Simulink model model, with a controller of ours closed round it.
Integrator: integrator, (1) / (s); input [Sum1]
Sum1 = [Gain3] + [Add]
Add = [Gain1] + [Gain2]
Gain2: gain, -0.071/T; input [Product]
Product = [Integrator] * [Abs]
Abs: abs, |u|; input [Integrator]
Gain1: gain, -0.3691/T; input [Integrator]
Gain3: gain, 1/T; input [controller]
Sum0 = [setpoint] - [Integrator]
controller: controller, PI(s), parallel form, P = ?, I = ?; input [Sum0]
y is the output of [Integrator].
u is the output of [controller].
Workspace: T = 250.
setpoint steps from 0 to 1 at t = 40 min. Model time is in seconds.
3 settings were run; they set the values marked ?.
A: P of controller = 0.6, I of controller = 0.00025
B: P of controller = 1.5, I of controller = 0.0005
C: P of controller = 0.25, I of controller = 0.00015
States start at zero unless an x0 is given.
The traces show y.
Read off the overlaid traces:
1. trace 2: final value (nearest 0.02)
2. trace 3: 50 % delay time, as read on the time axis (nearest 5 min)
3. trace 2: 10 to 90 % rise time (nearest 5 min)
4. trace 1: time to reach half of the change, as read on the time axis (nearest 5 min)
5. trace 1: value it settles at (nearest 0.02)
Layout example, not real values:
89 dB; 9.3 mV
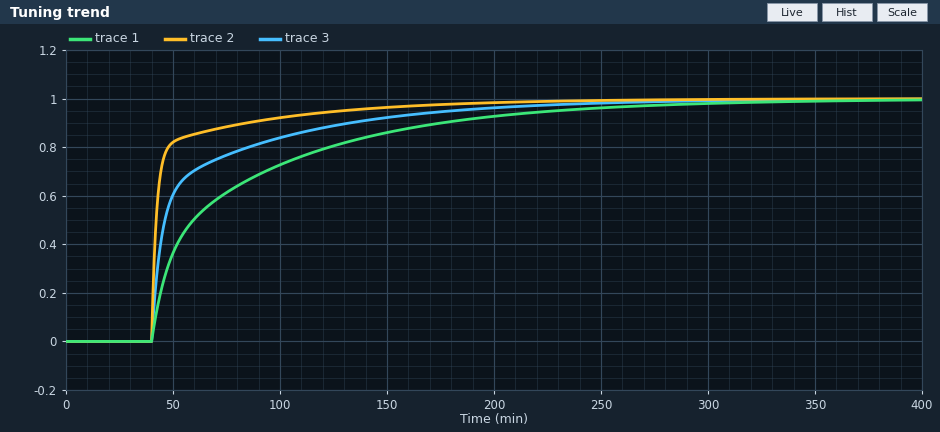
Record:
1.00; 45 min; 45 min; 60 min; 1.00
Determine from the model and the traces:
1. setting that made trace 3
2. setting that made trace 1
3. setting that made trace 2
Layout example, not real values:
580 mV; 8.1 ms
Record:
A; C; B
